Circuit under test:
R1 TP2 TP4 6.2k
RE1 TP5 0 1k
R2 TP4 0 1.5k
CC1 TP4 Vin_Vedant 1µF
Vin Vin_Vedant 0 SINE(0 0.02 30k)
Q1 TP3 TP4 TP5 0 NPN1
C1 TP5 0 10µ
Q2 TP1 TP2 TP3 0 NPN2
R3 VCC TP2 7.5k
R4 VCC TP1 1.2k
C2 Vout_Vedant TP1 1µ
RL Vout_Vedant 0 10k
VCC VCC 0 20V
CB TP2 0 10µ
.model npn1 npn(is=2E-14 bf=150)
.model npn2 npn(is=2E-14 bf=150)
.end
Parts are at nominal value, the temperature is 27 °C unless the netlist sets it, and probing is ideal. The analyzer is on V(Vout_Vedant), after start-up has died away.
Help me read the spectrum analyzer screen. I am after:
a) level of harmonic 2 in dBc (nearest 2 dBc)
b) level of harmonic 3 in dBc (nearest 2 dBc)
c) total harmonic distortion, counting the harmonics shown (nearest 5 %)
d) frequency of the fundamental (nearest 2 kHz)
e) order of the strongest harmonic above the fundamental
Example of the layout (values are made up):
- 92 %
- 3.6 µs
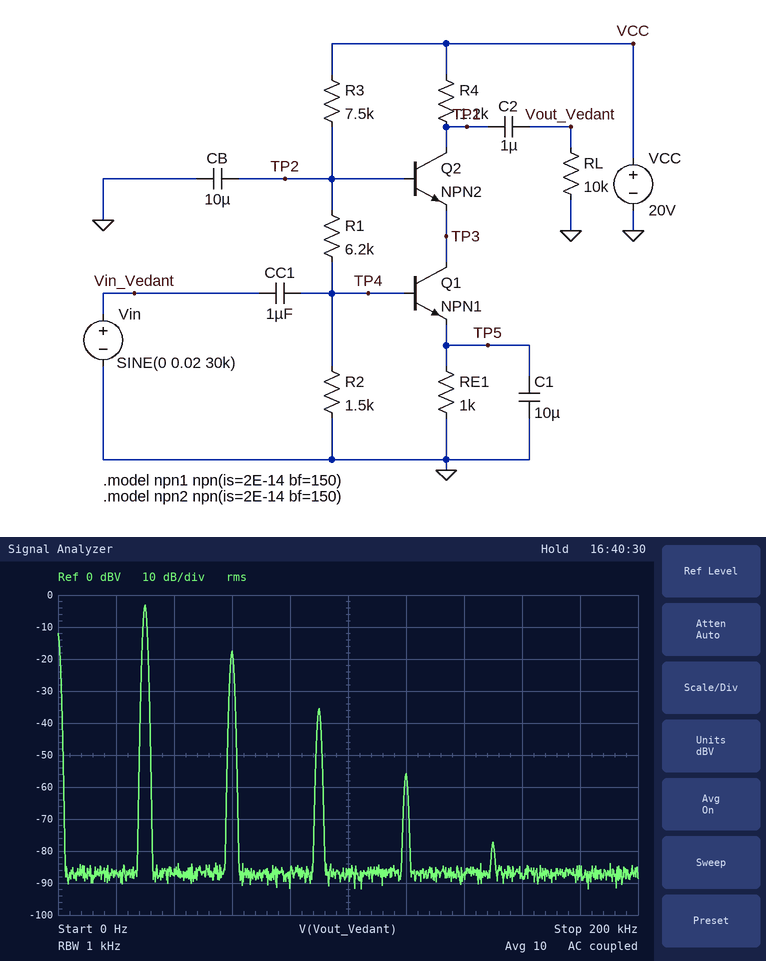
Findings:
- -14 dBc
- -32 dBc
- 20 %
- 30 kHz
- 2
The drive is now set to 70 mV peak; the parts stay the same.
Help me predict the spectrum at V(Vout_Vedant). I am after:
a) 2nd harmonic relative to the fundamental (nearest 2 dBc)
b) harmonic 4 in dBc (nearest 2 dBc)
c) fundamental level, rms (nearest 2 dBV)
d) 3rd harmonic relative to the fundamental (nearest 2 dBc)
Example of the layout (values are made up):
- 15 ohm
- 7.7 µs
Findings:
- -6 dBc
- -24 dBc
- 4 dBV
- -14 dBc
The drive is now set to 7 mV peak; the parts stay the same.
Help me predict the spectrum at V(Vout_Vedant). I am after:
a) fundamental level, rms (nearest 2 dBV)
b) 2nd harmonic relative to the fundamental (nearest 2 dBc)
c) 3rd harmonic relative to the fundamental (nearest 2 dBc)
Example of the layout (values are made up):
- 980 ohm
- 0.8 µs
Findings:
- -12 dBV
- -24 dBc
- -50 dBc
